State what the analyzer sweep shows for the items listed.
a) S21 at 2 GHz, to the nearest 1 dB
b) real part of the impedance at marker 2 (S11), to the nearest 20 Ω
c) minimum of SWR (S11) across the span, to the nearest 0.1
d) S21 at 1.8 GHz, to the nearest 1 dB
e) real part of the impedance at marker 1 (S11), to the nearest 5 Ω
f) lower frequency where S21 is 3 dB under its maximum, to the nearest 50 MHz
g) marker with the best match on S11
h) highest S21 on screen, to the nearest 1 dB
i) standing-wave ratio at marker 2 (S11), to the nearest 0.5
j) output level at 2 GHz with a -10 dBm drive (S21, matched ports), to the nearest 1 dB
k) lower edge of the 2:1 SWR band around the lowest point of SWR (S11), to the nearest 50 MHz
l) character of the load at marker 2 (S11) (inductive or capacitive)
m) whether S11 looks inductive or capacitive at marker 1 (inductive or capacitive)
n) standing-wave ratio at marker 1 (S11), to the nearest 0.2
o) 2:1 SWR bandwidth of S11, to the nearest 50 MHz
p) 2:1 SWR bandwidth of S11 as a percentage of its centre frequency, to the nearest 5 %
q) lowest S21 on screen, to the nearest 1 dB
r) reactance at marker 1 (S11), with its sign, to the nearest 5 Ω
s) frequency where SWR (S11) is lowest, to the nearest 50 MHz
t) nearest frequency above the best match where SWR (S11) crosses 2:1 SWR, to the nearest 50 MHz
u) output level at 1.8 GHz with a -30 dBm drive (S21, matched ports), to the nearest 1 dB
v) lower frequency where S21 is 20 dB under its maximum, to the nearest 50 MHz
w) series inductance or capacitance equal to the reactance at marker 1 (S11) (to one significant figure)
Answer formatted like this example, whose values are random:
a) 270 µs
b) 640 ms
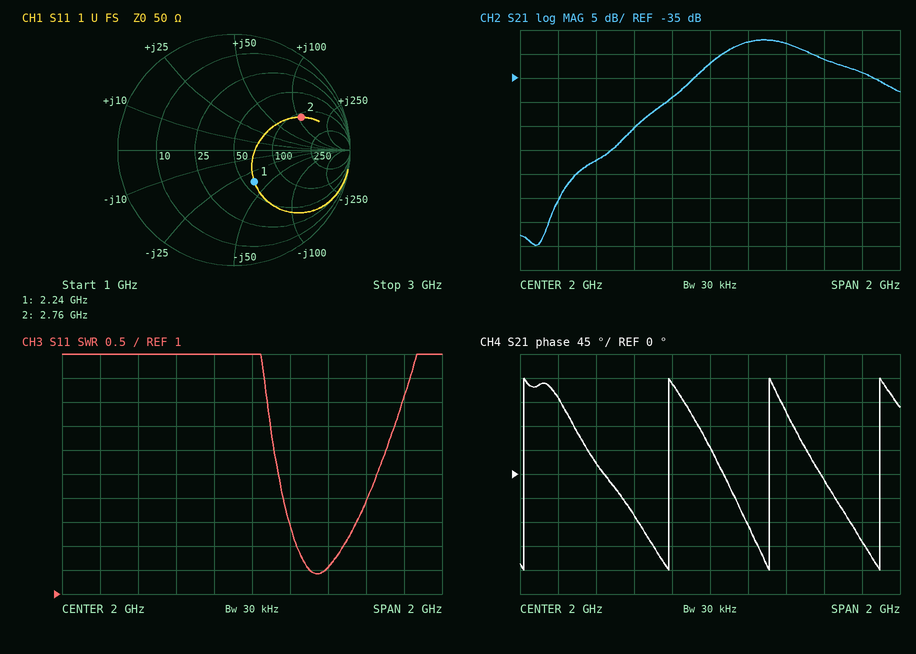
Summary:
a) -32 dB
b) 120 Ω
c) 1.4
d) -39 dB
e) 60 Ω
f) 2.05 GHz
g) marker 1
h) -27 dB
i) 4.5
j) -42 dBm
k) 2.25 GHz
l) inductive
m) capacitive
n) 2.0
o) 250 MHz
p) 10 %
q) -70 dB
r) -35 Ω
s) 2.35 GHz
t) 2.50 GHz
u) -69 dBm
v) 1.55 GHz
w) 2 pF
